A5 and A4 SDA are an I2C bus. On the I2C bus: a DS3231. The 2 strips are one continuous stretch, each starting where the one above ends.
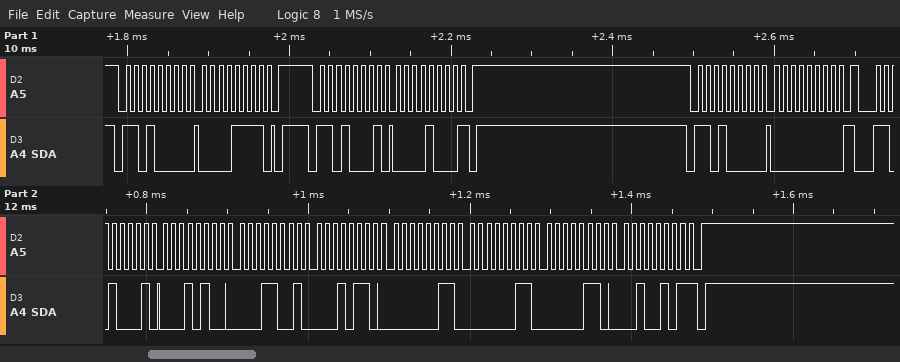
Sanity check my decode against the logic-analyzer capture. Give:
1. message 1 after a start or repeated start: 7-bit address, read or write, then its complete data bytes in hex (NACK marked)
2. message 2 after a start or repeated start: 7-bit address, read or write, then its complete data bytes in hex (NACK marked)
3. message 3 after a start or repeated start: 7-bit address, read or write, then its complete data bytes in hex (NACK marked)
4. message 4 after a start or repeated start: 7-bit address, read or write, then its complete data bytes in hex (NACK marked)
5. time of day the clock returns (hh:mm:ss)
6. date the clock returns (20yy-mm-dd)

0x68 write: 0F
0x68 read: 08 NACK
0x68 write: 00
0x68 read: 14 19 16 03 03 06 25 NACK
16:19:14
2025-06-03
